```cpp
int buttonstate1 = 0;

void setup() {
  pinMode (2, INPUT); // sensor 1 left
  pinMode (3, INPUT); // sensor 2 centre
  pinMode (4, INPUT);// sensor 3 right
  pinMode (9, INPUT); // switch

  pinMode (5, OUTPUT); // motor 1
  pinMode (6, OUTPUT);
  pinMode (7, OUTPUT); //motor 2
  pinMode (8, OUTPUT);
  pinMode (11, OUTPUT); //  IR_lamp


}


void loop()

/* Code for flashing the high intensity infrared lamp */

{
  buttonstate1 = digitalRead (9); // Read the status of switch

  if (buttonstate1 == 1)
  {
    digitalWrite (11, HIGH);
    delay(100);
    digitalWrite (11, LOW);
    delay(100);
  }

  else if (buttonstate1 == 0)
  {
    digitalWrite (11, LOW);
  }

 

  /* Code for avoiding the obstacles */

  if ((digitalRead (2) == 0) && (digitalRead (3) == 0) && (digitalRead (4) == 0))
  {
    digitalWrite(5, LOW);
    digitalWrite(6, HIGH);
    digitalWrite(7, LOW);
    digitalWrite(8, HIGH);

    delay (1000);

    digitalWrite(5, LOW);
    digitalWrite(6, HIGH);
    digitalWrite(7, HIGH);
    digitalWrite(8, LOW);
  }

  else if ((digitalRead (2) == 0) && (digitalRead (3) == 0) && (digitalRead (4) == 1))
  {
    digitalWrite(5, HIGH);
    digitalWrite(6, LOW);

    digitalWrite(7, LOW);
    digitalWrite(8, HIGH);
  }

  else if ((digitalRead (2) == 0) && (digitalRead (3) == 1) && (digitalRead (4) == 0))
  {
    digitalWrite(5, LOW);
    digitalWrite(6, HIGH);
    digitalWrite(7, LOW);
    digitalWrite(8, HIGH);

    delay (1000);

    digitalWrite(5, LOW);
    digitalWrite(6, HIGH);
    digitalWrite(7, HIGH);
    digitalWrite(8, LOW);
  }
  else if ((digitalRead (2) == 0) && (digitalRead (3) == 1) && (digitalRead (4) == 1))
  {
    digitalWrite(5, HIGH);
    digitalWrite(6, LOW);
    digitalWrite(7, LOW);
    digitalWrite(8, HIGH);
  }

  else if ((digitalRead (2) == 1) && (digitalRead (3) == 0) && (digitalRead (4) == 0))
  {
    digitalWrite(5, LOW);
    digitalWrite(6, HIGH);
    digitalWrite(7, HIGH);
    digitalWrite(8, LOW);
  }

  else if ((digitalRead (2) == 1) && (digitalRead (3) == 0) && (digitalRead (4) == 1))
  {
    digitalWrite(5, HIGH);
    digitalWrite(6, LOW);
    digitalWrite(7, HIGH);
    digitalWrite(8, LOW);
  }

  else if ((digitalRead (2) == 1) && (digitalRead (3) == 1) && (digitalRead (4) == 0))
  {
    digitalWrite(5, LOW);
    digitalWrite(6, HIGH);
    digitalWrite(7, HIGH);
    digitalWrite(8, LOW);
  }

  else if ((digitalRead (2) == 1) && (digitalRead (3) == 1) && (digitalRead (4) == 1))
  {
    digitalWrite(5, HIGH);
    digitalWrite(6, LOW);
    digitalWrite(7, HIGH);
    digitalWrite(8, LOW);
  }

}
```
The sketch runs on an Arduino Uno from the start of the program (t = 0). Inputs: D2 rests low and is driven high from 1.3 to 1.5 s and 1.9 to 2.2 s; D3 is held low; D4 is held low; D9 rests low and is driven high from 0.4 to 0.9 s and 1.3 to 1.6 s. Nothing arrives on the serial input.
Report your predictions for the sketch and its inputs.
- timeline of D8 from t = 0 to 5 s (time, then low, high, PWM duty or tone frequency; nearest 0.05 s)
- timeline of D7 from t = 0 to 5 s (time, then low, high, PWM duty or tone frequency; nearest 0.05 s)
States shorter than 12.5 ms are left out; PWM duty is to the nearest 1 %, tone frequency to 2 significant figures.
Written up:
0 s high; 2 s low; 2.2 s high
0 s low; 2 s high; 2.2 s low
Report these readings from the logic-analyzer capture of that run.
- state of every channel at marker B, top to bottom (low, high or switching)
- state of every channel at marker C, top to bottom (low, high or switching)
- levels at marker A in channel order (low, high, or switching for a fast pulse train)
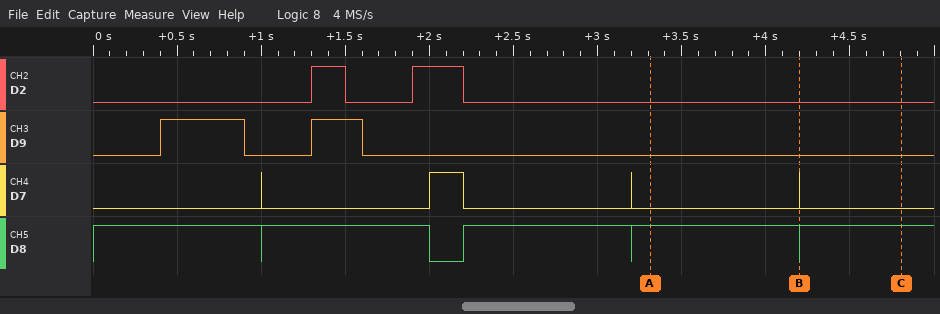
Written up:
D2 low, D9 low, D7 low, D8 high
D2 low, D9 low, D7 low, D8 high
D2 low, D9 low, D7 low, D8 high
